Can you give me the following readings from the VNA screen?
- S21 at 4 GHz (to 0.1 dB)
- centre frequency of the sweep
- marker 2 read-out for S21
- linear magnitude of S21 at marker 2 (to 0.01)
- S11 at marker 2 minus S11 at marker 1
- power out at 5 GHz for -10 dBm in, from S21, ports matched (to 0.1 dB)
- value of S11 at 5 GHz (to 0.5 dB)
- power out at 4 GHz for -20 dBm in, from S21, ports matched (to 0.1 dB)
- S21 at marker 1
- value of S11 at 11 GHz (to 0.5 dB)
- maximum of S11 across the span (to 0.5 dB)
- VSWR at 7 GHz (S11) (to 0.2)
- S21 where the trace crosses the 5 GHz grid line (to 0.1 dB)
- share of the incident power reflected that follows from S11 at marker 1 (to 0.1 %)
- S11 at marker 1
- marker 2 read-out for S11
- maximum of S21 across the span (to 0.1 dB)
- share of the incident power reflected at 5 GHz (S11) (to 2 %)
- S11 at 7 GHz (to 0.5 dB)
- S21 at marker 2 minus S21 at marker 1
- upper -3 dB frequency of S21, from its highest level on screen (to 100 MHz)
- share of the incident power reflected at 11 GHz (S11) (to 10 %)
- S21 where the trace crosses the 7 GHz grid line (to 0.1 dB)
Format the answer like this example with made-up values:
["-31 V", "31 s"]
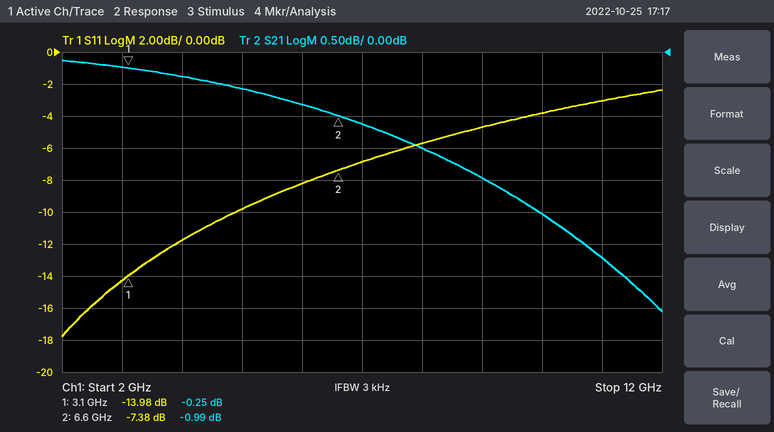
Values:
["-0.4 dB", "7 GHz", "-0.99 dB", "0.89", "6.60 dB", "-10.6 dBm", "-10.0 dB", "-20.4 dBm", "-0.25 dB", "-3.0 dB", "-2.5 dB", "2.6", "-0.6 dB", "4.0 %", "-13.98 dB", "-7.38 dB", "-0.1 dB", "10 %", "-7.0 dB", "-0.74 dB", "10.9 GHz", "50 %", "-1.1 dB"]
